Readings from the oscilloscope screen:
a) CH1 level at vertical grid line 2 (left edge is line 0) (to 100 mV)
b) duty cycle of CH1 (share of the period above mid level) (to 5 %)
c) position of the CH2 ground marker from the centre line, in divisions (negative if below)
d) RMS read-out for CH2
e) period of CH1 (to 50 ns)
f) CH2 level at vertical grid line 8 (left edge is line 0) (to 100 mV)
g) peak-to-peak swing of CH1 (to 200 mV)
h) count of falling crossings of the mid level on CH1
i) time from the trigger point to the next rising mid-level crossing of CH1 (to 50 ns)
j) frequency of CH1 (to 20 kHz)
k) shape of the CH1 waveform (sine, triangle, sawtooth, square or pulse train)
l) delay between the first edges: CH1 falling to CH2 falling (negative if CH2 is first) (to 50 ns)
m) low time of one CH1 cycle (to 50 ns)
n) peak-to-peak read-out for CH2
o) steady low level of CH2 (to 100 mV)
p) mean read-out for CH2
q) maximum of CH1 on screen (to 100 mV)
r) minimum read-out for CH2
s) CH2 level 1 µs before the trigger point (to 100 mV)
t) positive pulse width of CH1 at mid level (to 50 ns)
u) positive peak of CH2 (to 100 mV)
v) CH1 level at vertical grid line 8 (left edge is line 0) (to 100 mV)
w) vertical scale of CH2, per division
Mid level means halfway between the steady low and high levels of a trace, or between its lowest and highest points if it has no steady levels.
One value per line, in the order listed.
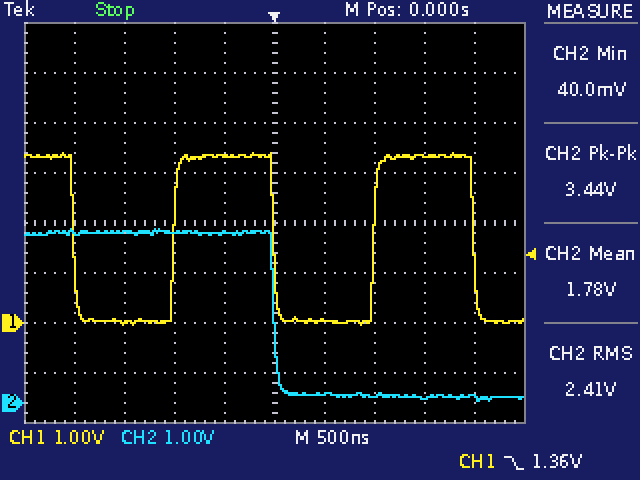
0.0 V
50 %
-3.6 div
2.41 V
2.00 µs
100 mV
3.4 V
3
1.00 µs
500 kHz
square
+2.00 µs
1.00 µs
3.44 V
100 mV
1.78 V
3.4 V
40.0 mV
3.4 V
1.00 µs
3.5 V
3.3 V
1 V
